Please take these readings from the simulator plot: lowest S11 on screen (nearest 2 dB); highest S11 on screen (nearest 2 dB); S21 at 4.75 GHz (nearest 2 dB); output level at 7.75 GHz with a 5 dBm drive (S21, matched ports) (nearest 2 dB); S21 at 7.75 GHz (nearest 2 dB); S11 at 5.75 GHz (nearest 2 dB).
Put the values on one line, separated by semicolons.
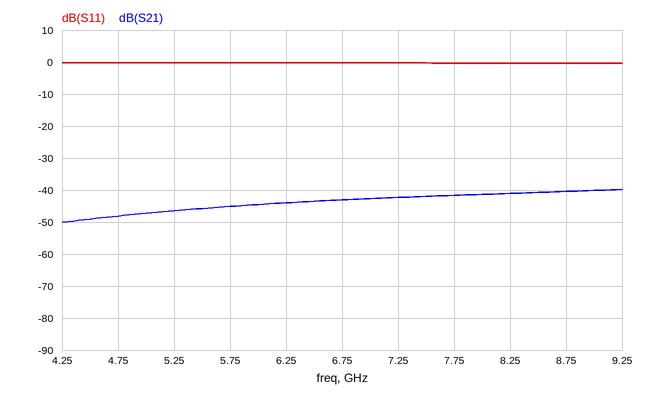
0 dB; 0 dB; -48 dB; -36 dBm; -42 dB; 0 dB
